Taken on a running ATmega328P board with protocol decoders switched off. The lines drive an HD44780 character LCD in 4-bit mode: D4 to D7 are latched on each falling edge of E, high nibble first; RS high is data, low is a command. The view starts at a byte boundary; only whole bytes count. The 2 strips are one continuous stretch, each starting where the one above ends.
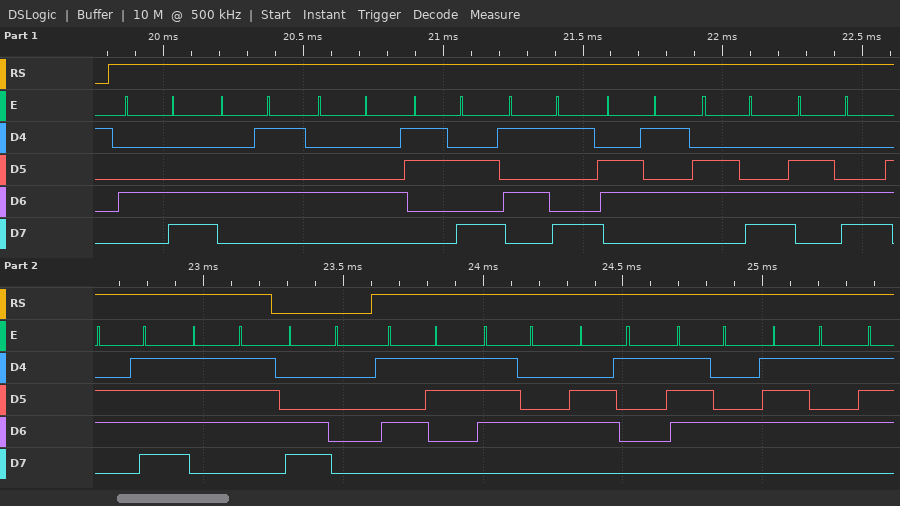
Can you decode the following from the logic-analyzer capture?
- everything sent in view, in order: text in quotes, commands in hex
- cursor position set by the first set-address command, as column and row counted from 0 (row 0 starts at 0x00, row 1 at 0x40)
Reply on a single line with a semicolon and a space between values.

"LED:Yellow" 0xC0 "Statu"; column 0, row 1
